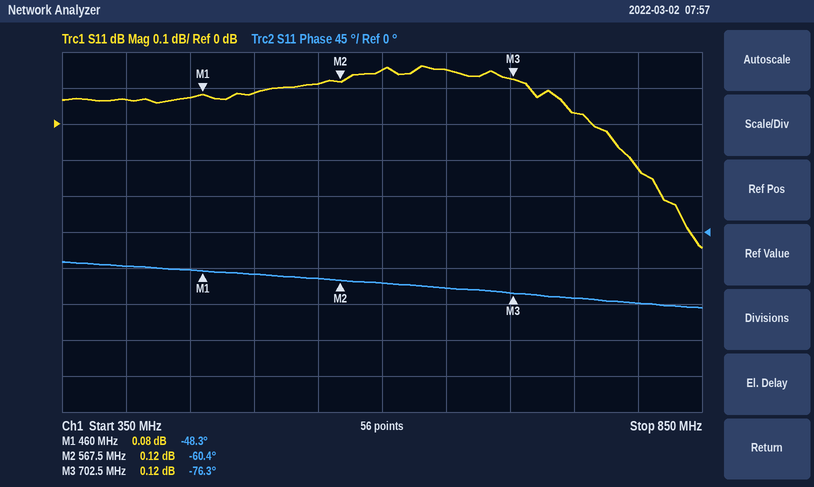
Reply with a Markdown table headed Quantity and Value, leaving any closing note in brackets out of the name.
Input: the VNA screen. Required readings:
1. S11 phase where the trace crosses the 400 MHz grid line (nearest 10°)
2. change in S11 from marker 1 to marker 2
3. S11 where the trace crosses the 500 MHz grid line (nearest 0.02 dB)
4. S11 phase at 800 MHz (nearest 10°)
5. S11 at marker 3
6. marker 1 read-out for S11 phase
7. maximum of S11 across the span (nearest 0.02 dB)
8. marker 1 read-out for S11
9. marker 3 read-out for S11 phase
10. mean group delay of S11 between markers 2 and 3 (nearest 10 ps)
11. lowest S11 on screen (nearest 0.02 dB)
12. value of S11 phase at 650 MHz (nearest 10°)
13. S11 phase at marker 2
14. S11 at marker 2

| Quantity | Value |
|---|---|
| S11 phase where the trace crosses the 400 MHz grid line | -40° |
| change in S11 from marker 1 to marker 2 | 0.04 dB |
| S11 where the trace crosses the 500 MHz grid line | 0.08 dB |
| S11 phase at 800 MHz | -90° |
| S11 at marker 3 | 0.12 dB |
| marker 1 read-out for S11 phase | -48.3° |
| maximum of S11 across the span | 0.16 dB |
| marker 1 read-out for S11 | 0.08 dB |
| marker 3 read-out for S11 phase | -76.3° |
| mean group delay of S11 between markers 2 and 3 | 330 ps |
| lowest S11 on screen | -0.34 dB |
| value of S11 phase at 650 MHz | -70° |
| S11 phase at marker 2 | -60.4° |
| S11 at marker 2 | 0.12 dB |
